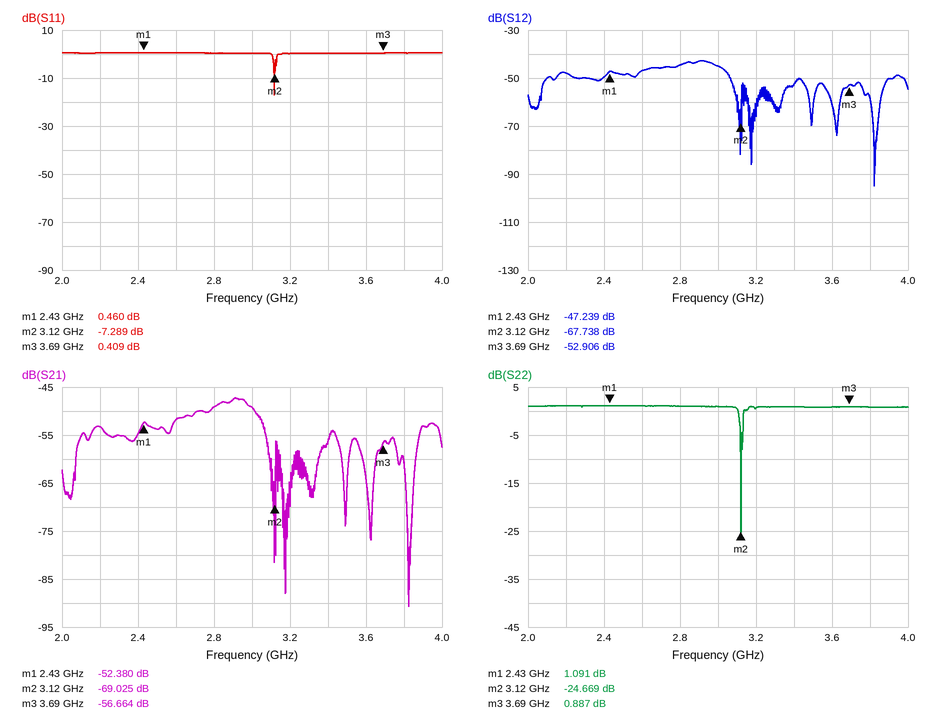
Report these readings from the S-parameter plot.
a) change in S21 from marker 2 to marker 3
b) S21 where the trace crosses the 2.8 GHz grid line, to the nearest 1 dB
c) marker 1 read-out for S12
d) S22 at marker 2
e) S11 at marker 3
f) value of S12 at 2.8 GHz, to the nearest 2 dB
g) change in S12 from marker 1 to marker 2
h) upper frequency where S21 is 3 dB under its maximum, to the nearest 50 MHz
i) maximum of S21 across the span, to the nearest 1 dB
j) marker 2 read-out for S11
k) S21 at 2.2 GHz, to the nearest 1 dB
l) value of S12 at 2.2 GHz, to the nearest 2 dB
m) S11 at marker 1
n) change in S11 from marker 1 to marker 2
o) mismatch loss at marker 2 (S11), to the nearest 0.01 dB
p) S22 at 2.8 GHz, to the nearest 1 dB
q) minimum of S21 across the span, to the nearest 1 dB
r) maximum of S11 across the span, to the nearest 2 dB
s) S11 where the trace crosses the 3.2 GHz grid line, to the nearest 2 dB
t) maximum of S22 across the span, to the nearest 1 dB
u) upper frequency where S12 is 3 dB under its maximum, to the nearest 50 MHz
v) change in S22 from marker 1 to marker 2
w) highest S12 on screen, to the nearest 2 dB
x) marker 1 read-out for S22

12.361 dB
-49 dB
-47.239 dB
-24.669 dB
0.409 dB
-44 dB
-20.499 dB
3.00 GHz
-47 dB
-7.289 dB
-53 dB
-48 dB
0.460 dB
-7.749 dB
0.90 dB
1 dB
-91 dB
0 dB
0 dB
1 dB
3.00 GHz
-25.760 dB
-42 dB
1.091 dB
